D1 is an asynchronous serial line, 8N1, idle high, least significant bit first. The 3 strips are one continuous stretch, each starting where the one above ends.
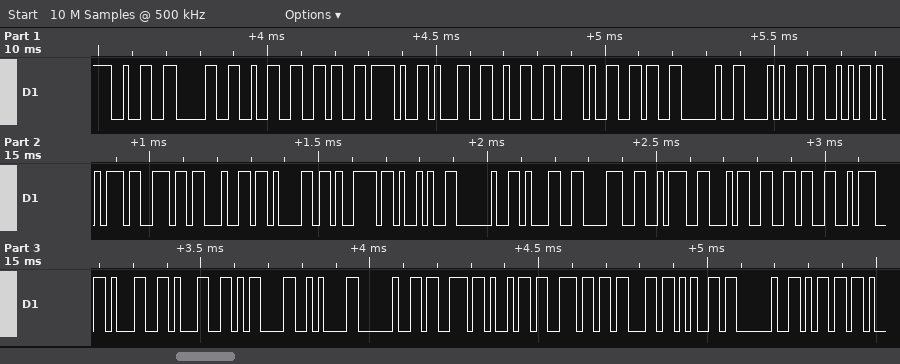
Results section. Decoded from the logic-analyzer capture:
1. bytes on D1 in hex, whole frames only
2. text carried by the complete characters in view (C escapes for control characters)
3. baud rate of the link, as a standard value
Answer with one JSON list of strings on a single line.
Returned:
["32 30 32 36 2F 31 32 2F 36 20 28 53 75 6E 64 61 79 29 20 31 38 3A 34 36 3A 31 31 0D 0A 20 73 69 6E 63 65 20 6D", "\"2026/12/6 (Sunday) 18:46:11\\r\\n since m\"", "57600 baud"]
